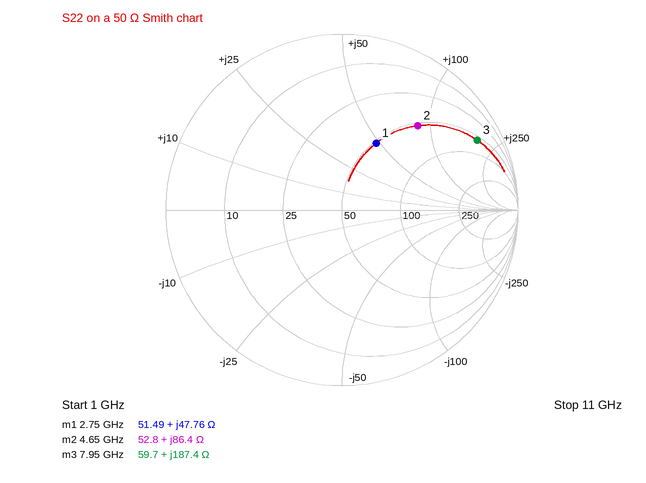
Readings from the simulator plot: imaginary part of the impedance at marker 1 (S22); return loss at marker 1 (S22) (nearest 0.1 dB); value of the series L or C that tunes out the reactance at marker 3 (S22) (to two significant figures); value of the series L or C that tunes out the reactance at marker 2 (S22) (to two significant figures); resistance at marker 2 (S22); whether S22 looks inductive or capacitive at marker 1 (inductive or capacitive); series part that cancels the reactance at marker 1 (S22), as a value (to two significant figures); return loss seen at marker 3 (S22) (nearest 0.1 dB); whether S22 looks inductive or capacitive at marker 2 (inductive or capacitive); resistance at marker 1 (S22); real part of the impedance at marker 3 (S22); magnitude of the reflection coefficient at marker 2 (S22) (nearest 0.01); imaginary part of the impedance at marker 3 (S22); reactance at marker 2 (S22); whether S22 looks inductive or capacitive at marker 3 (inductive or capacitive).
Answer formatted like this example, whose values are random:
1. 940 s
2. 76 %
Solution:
1. +47.76 Ω
2. 7.4 dB
3. 110 fF
4. 400 fF
5. 52.8 Ω
6. inductive
7. 1.2 pF
8. 1.3 dB
9. inductive
10. 51.49 Ω
11. 59.7 Ω
12. 0.64
13. +187.4 Ω
14. +86.4 Ω
15. inductive
